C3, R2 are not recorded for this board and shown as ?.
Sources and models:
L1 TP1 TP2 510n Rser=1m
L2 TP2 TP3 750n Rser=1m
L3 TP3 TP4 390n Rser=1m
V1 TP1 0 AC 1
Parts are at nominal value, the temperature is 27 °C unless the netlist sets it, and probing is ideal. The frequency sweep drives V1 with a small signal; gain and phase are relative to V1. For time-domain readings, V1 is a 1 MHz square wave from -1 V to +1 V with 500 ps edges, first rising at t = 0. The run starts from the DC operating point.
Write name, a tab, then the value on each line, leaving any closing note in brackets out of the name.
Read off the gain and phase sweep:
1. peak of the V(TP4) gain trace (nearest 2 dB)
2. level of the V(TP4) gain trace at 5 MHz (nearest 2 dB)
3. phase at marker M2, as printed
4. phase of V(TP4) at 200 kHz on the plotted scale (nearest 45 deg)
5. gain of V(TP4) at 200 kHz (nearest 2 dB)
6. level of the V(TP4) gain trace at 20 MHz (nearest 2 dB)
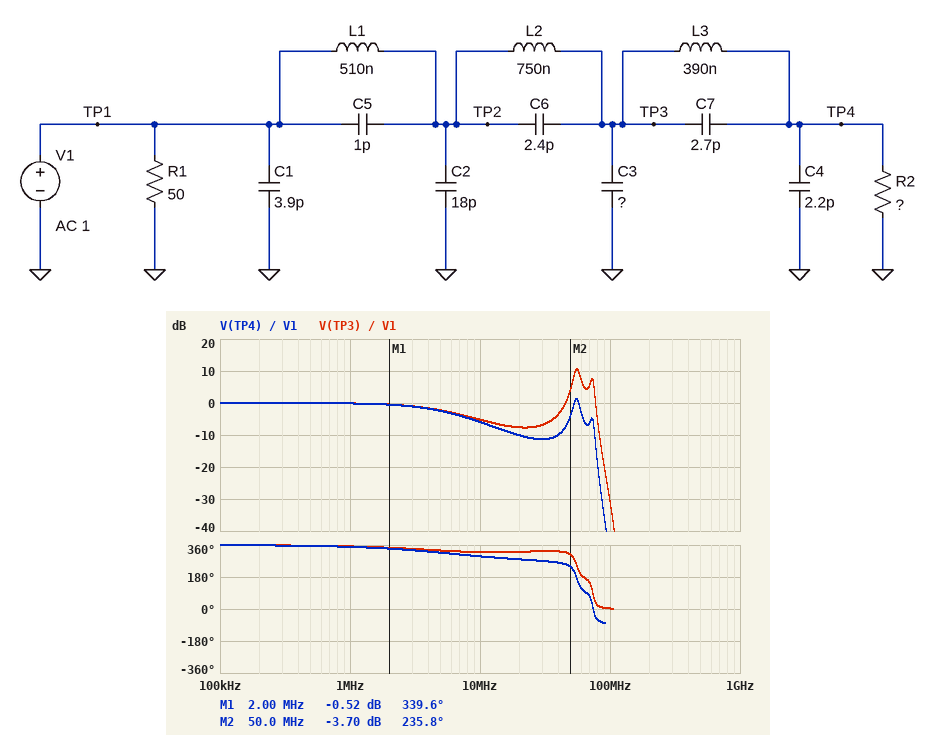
peak of the V(TP4) gain trace	2 dB
level of the V(TP4) gain trace at 5 MHz	-2 dB
phase at marker M2, as printed	235.8 deg
phase of V(TP4) at 200 kHz on the plotted scale	360 deg
gain of V(TP4) at 200 kHz	0 dB
level of the V(TP4) gain trace at 20 MHz	-10 dB
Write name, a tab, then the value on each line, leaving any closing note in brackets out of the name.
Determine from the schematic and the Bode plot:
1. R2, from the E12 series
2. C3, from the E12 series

R2, from the E12 series	56 Ω
C3, from the E12 series	15 pF
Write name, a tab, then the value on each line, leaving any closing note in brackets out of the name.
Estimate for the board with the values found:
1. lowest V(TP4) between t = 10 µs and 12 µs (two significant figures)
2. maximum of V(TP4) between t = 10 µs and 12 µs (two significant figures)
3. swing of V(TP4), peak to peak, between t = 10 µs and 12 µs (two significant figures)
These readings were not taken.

lowest V(TP4) between t = 10 µs and 12 µs	-1.0 V
maximum of V(TP4) between t = 10 µs and 12 µs	1.0 V
swing of V(TP4), peak to peak, between t = 10 µs and 12 µs	2.0 V
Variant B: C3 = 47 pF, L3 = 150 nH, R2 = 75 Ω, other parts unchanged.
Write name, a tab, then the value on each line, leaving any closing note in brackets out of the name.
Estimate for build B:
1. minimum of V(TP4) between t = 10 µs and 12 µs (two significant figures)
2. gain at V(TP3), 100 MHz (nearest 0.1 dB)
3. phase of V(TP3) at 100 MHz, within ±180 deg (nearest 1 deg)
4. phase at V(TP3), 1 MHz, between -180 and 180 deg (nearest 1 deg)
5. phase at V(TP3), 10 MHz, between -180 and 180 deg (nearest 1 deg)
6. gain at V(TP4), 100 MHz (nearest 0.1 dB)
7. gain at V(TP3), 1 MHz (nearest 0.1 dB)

minimum of V(TP4) between t = 10 µs and 12 µs	-1.1 V
gain at V(TP3), 100 MHz	-41.8 dB
phase of V(TP3) at 100 MHz, within ±180 deg	11 deg
phase at V(TP3), 1 MHz, between -180 and 180 deg	-6 deg
phase at V(TP3), 10 MHz, between -180 and 180 deg	-50 deg
gain at V(TP4), 100 MHz	-46.5 dB
gain at V(TP3), 1 MHz	0 dB
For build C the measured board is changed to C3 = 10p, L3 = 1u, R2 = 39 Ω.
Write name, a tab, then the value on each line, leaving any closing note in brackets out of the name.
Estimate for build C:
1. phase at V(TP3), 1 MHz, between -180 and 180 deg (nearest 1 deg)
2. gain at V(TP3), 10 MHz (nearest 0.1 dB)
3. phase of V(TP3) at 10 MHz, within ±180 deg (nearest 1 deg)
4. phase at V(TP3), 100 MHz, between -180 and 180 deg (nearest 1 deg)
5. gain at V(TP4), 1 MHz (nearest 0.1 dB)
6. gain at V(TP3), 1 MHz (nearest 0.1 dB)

phase at V(TP3), 1 MHz, between -180 and 180 deg	-11 deg
gain at V(TP3), 10 MHz	-5.5 dB
phase of V(TP3) at 10 MHz, within ±180 deg	-17 deg
phase at V(TP3), 100 MHz, between -180 and 180 deg	0 deg
gain at V(TP4), 1 MHz	-0.5 dB
gain at V(TP3), 1 MHz	-0.4 dB
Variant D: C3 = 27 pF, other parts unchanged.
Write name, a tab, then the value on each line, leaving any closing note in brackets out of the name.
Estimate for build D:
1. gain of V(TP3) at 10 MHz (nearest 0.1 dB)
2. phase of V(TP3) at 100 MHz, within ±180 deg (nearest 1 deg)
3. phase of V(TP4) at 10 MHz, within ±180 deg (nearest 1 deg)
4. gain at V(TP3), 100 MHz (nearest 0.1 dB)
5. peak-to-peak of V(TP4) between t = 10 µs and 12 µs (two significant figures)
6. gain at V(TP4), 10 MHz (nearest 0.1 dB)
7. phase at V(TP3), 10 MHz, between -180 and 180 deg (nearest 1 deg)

gain of V(TP3) at 10 MHz	-5.0 dB
phase of V(TP3) at 100 MHz, within ±180 deg	1 deg
phase of V(TP4) at 10 MHz, within ±180 deg	-65 deg
gain at V(TP3), 100 MHz	-37.5 dB
peak-to-peak of V(TP4) between t = 10 µs and 12 µs	2.1 V
gain at V(TP4), 10 MHz	-5.7 dB
phase at V(TP3), 10 MHz, between -180 and 180 deg	-41 deg
